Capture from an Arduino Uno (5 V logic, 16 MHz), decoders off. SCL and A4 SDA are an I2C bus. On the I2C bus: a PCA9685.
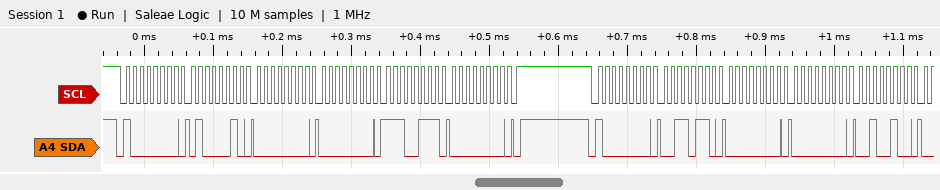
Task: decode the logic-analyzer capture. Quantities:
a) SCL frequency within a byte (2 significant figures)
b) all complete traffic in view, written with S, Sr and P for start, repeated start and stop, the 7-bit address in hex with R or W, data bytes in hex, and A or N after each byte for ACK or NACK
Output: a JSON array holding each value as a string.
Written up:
["100 kHz", "S 40W A 42 A 00 A 00 A E7 A 00 A P S 40W A 36 A 00 A 00 A 24 A"]
